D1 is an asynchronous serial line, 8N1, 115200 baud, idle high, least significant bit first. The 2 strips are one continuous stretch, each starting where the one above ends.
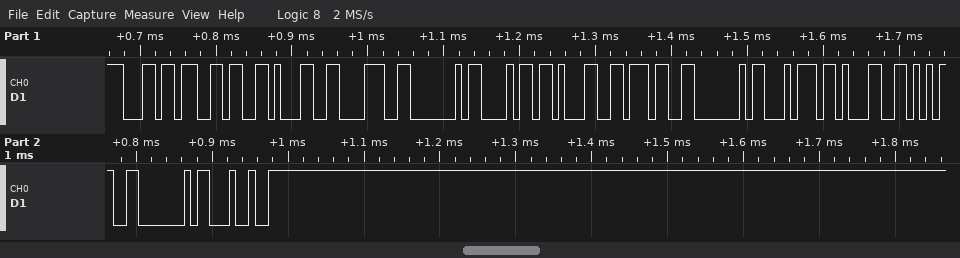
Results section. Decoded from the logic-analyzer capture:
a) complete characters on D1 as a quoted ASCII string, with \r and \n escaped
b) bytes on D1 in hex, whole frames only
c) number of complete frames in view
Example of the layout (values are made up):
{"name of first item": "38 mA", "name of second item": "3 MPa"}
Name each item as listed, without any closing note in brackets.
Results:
{"complete characters on D1 as a quoted ASCII string, with \\r and \\n escaped": "\"l618@h17@t15@$\"", "bytes on D1 in hex, whole frames only": "6C 36 31 38 40 68 31 37 40 74 31 35 40 24", "number of complete frames in view": "14"}
